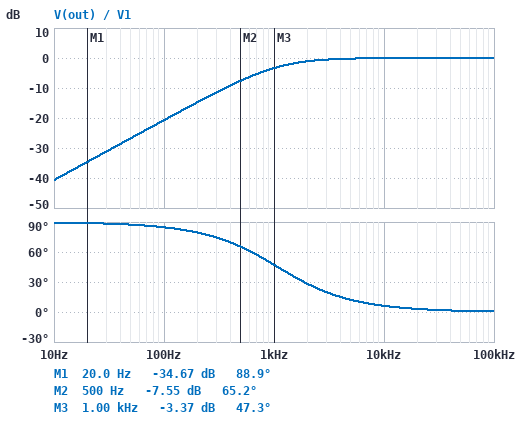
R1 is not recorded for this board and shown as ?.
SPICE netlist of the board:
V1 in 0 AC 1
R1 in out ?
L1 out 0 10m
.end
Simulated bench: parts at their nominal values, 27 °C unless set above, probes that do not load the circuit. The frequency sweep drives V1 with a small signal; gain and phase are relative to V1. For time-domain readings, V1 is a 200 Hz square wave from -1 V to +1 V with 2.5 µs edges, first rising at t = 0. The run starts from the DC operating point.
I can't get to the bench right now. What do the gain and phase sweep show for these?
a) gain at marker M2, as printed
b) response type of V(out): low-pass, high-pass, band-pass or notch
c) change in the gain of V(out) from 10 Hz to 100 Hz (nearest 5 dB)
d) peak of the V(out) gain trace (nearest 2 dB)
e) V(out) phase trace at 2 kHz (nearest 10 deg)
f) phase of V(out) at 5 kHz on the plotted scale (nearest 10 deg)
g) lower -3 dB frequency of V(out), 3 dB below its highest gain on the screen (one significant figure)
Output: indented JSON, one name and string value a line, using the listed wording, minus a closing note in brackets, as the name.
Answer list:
{
  "gain at marker M2, as printed": "-7.55 dB",
  "response type of V(out): low-pass, high-pass, band-pass or notch": "high-pass",
  "change in the gain of V(out) from 10 Hz to 100 Hz": "20 dB",
  "peak of the V(out) gain trace": "0 dB",
  "V(out) phase trace at 2 kHz": "30 deg",
  "phase of V(out) at 5 kHz on the plotted scale": "10 deg",
  "lower -3 dB frequency of V(out), 3 dB below its highest gain on the screen": "1 kHz"
}
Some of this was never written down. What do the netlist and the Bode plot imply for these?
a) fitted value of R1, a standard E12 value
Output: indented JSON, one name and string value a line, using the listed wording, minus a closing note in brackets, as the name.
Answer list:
{
  "fitted value of R1, a standard E12 value": "68 Ω"
}
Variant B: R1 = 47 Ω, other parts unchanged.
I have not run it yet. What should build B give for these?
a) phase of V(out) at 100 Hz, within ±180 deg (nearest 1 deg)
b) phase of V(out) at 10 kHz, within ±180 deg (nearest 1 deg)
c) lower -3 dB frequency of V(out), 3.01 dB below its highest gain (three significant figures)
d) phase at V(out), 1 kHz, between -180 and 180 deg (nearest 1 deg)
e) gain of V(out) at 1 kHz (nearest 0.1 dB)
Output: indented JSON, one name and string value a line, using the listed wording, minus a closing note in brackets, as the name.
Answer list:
{
  "phase of V(out) at 100 Hz, within ±180 deg": "82 deg",
  "phase of V(out) at 10 kHz, within ±180 deg": "4 deg",
  "lower -3 dB frequency of V(out), 3.01 dB below its highest gain": "748 Hz",
  "phase at V(out), 1 kHz, between -180 and 180 deg": "37 deg",
  "gain of V(out) at 1 kHz": "-1.9 dB"
}
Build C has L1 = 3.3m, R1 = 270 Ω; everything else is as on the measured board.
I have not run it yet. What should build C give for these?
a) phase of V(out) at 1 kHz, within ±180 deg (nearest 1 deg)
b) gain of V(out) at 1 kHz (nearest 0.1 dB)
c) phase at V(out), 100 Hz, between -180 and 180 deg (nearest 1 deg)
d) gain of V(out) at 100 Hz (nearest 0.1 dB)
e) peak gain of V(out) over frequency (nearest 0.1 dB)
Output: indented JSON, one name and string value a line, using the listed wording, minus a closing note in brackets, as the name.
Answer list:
{
  "phase of V(out) at 1 kHz, within ±180 deg": "86 deg",
  "gain of V(out) at 1 kHz": "-22.3 dB",
  "phase at V(out), 100 Hz, between -180 and 180 deg": "90 deg",
  "gain of V(out) at 100 Hz": "-42.3 dB",
  "peak gain of V(out) over frequency": "0 dB"
}
